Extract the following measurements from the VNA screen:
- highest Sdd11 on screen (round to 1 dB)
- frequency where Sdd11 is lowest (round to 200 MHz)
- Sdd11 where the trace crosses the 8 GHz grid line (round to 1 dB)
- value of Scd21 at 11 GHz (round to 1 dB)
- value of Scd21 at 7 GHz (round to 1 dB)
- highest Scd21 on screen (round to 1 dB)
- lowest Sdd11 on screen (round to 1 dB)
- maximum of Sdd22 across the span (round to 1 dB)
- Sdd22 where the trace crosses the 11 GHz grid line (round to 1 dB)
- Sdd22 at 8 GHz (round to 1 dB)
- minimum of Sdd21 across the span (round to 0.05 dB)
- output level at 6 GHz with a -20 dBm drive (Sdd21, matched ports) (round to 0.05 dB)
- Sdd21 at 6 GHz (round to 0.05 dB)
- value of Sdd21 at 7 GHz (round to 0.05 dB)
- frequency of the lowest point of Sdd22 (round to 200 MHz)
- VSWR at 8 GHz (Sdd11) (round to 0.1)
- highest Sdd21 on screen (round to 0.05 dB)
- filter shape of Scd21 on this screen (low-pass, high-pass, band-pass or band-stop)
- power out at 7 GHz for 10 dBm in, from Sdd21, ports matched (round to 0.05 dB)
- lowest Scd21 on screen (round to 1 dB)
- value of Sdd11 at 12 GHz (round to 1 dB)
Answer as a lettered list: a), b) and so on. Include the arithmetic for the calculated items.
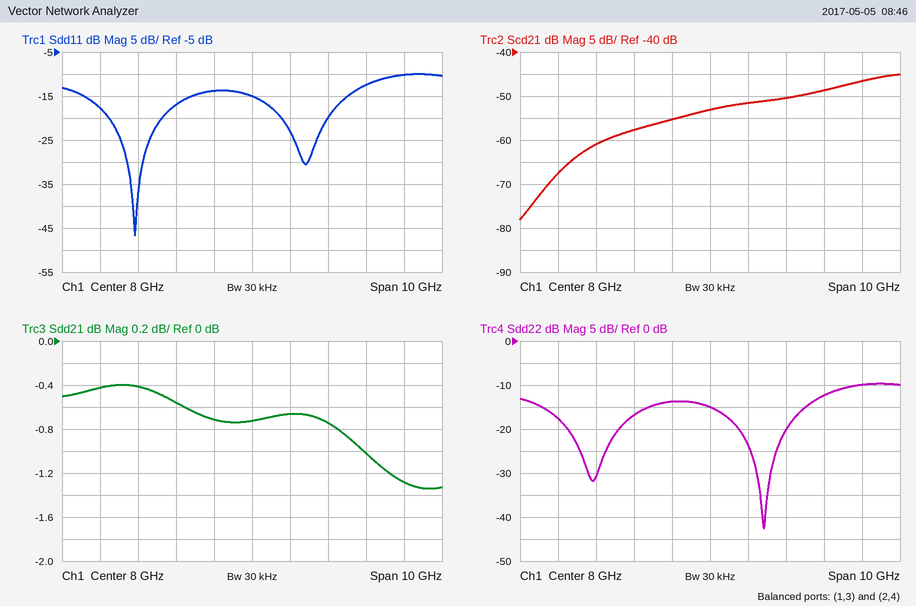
a) -10 dB
b) 5.0 GHz
c) -15 dB
d) -49 dB
e) -55 dB
f) -45 dB
g) -47 dB
h) -10 dB
i) -12 dB
j) -15 dB
k) -1.35 dB
l) -20 dBm + (-0.55 dB) = -20.55 dBm
m) -0.55 dB
n) -0.70 dB
o) 9.4 GHz
p) |Γ| = 10^(-15/20) = 0.1778; VSWR = (1 + 0.1778)/(1 − 0.1778) ≈ 1.4
q) -0.40 dB
r) high-pass
s) 10 dBm + (-0.70 dB) = 9.30 dBm
t) -78 dB
u) -10 dB
